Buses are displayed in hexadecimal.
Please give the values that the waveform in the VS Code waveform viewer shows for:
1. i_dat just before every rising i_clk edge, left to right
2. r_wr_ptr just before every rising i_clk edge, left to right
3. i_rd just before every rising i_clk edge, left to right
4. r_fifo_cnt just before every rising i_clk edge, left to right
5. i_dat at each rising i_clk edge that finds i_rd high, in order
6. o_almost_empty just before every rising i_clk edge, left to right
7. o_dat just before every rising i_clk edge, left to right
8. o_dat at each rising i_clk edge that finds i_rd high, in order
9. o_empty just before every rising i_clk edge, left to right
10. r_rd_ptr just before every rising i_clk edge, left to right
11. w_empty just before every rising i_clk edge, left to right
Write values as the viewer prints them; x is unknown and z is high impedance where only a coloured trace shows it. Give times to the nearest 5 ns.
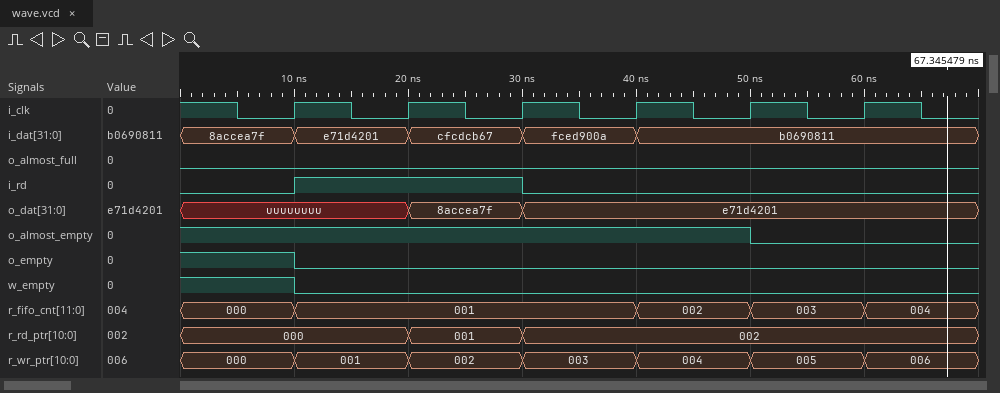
8accea7f, e71d4201, cfcdcb67, fced900a, b0690811, b0690811
000, 001, 002, 003, 004, 005
0 1 1 0 0 0
000, 001, 001, 001, 002, 003
e71d4201, cfcdcb67
1 1 1 1 1 0
uuuuuuuu, uuuuuuuu, 8accea7f, e71d4201, e71d4201, e71d4201
uuuuuuuu, 8accea7f
1 0 0 0 0 0
000, 000, 001, 002, 002, 002
1 0 0 0 0 0
